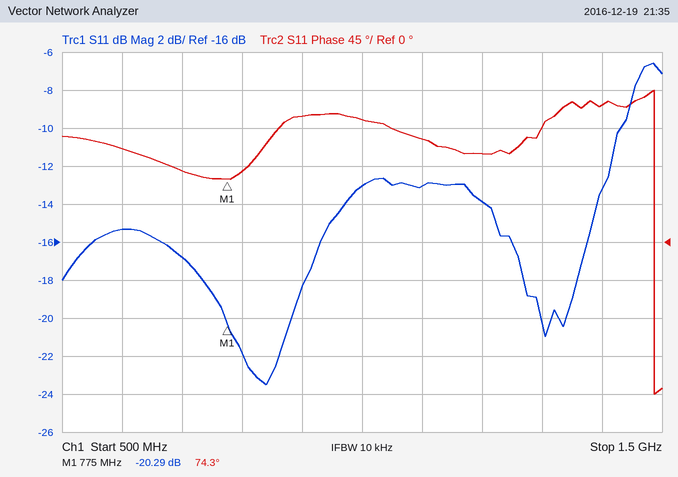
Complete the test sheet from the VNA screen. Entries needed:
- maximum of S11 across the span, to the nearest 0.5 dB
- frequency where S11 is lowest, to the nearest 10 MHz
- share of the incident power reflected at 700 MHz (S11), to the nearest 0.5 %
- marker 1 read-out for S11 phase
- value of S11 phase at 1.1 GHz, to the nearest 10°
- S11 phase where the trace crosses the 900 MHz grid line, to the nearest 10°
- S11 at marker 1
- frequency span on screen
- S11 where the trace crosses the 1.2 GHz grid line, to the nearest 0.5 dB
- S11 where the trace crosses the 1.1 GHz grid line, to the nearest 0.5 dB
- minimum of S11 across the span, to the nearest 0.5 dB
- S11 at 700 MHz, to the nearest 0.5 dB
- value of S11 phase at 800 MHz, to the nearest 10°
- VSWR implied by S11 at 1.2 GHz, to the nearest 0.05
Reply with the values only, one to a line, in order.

-6.5 dB
840 MHz
2.0 %
74.3°
120°
150°
-20.29 dB
1 GHz
-14.0 dB
-13.0 dB
-23.5 dB
-17.0 dB
80°
1.50
